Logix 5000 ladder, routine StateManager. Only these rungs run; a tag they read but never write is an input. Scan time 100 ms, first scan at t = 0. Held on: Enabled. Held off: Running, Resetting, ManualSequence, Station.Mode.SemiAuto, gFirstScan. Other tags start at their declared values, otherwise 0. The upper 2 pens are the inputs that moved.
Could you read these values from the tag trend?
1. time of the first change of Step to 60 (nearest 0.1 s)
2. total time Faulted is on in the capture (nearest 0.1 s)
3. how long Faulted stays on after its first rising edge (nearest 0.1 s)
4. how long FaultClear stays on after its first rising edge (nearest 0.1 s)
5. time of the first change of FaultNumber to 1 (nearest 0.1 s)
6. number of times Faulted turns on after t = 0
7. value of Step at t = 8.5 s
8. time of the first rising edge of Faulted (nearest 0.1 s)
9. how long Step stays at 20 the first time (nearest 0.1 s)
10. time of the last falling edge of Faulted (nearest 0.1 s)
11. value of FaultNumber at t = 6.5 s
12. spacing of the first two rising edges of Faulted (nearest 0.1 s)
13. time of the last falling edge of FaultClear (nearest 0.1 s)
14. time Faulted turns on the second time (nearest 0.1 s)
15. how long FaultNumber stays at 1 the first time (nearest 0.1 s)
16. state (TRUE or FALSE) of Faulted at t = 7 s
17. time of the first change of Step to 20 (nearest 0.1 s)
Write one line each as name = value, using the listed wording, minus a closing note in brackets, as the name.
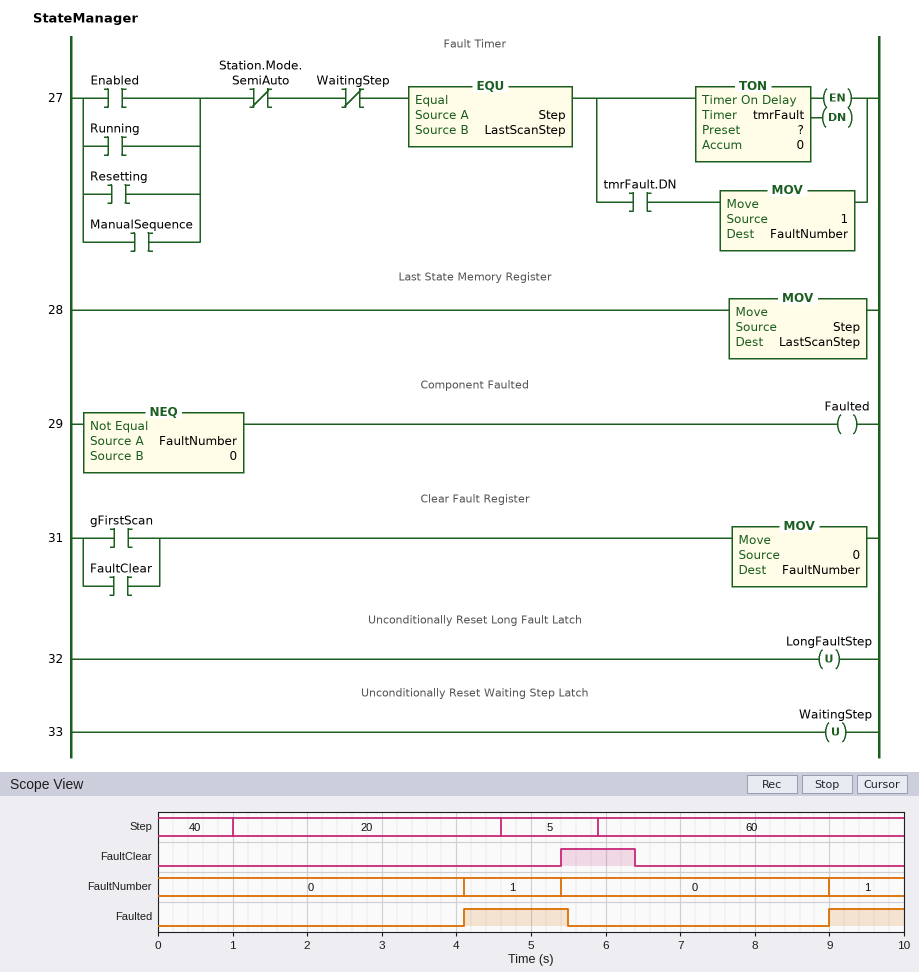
time of the first change of Step to 60 = 5.9 s
total time Faulted is on in the capture = 2.4 s
how long Faulted stays on after its first rising edge = 1.4 s
how long FaultClear stays on after its first rising edge = 1.0 s
time of the first change of FaultNumber to 1 = 4.1 s
number of times Faulted turns on after t = 0 = 2
value of Step at t = 8.5 s = 60
time of the first rising edge of Faulted = 4.1 s
how long Step stays at 20 the first time = 3.6 s
time of the last falling edge of Faulted = 5.5 s
value of FaultNumber at t = 6.5 s = 0
spacing of the first two rising edges of Faulted = 4.9 s
time of the last falling edge of FaultClear = 6.4 s
time Faulted turns on the second time = 9.0 s
how long FaultNumber stays at 1 the first time = 1.3 s
state (TRUE or FALSE) of Faulted at t = 7 s = FALSE
time of the first change of Step to 20 = 1.0 s
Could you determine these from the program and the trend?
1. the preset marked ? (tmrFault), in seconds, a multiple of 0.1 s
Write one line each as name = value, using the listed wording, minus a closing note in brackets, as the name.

the preset marked ? (tmrFault), in seconds, a multiple of 0.1 s = 3.0 s
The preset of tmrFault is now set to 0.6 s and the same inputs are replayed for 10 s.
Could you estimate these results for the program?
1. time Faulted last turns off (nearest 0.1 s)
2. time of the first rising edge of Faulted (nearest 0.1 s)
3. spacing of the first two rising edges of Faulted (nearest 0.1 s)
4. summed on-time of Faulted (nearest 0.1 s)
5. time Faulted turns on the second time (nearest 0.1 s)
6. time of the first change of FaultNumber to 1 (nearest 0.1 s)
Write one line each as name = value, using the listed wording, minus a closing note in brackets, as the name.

time Faulted last turns off = 5.9 s
time of the first rising edge of Faulted = 0.7 s
spacing of the first two rising edges of Faulted = 5.9 s
summed on-time of Faulted = 8.6 s
time Faulted turns on the second time = 6.6 s
time of the first change of FaultNumber to 1 = 0.7 s
